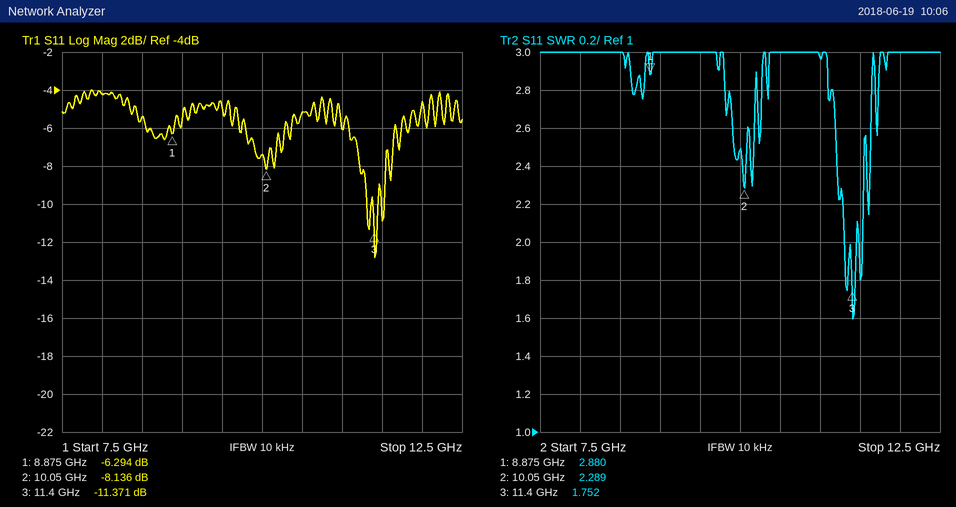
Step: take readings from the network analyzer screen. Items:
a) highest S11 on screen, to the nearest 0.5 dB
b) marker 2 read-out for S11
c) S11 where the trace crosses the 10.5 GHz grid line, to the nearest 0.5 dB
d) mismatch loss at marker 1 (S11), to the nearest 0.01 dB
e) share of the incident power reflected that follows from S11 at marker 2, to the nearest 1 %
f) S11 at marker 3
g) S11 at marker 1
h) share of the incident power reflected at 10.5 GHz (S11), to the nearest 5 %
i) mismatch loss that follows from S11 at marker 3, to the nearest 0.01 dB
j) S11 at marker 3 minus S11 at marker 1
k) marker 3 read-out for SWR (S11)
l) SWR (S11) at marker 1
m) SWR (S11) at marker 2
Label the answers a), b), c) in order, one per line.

a) -4.0 dB
b) -8.136 dB
c) -5.0 dB
d) 1.16 dB
e) 15 %
f) -11.371 dB
g) -6.294 dB
h) 30 %
i) 0.33 dB
j) -5.077 dB
k) 1.752
l) 2.880
m) 2.289
